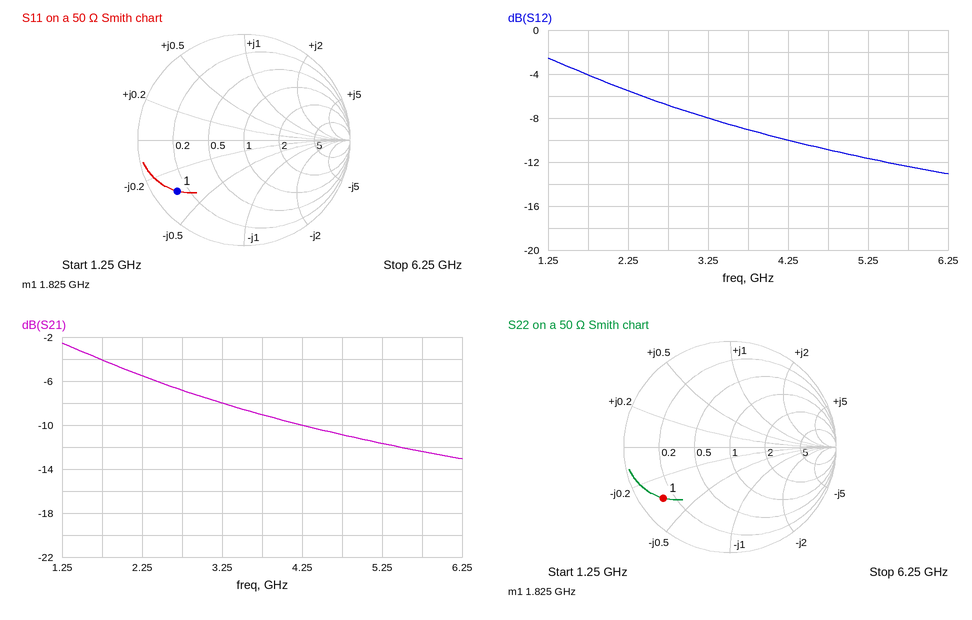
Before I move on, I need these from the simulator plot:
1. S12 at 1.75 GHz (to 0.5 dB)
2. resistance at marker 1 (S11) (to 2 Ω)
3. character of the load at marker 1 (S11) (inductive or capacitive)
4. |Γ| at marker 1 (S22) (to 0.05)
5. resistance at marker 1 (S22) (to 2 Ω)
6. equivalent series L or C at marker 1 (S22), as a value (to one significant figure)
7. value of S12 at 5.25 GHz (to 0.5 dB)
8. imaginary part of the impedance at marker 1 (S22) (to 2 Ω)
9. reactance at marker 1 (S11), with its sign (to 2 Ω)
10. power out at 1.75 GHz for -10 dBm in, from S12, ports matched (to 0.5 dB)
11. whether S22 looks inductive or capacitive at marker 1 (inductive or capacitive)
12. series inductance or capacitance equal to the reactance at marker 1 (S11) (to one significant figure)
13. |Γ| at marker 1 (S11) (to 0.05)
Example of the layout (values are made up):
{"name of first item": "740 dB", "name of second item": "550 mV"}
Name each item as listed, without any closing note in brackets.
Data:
{"S12 at 1.75 GHz": "-4.0 dB", "resistance at marker 1 (S11)": "6 Ω", "character of the load at marker 1 (S11)": "capacitive", "|Γ| at marker 1 (S22)": "0.80", "resistance at marker 1 (S22)": "6 Ω", "equivalent series L or C at marker 1 (S22), as a value": "5 pF", "value of S12 at 5.25 GHz": "-11.5 dB", "imaginary part of the impedance at marker 1 (S22)": "-16 Ω", "reactance at marker 1 (S11), with its sign": "-16 Ω", "power out at 1.75 GHz for -10 dBm in, from S12, ports matched": "-14.0 dBm", "whether S22 looks inductive or capacitive at marker 1": "capacitive", "series inductance or capacitance equal to the reactance at marker 1 (S11)": "5 pF", "|Γ| at marker 1 (S11)": "0.80"}
